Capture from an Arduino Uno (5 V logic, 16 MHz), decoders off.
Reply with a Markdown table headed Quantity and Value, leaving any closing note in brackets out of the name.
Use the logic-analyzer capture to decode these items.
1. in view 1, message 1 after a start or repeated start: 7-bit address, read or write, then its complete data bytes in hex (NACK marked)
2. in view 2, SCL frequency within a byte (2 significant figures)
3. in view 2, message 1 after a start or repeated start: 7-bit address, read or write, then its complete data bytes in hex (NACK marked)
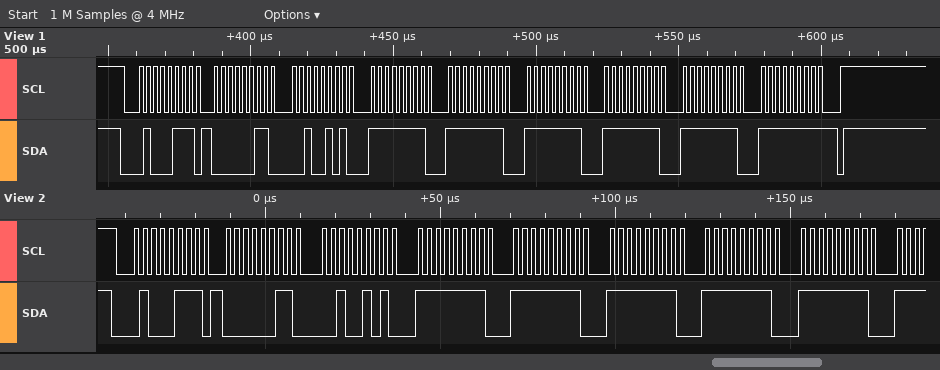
| Quantity | Value |
|---|---|
| in view 1, message 1 after a start or repeated start: 7-bit address, read or write, then its complete data bytes in hex | 0x23 read: 03 25 FF FF FF FF FF FF NACK |
| in view 2, SCL frequency within a byte | 400 kHz |
| in view 2, message 1 after a start or repeated start: 7-bit address, read or write, then its complete data bytes in hex | 0x23 read: 03 25 FF FF FF FF FF |
